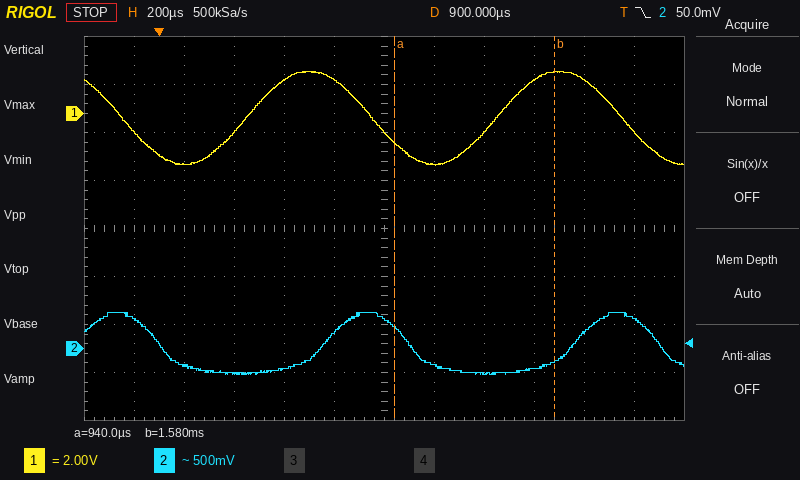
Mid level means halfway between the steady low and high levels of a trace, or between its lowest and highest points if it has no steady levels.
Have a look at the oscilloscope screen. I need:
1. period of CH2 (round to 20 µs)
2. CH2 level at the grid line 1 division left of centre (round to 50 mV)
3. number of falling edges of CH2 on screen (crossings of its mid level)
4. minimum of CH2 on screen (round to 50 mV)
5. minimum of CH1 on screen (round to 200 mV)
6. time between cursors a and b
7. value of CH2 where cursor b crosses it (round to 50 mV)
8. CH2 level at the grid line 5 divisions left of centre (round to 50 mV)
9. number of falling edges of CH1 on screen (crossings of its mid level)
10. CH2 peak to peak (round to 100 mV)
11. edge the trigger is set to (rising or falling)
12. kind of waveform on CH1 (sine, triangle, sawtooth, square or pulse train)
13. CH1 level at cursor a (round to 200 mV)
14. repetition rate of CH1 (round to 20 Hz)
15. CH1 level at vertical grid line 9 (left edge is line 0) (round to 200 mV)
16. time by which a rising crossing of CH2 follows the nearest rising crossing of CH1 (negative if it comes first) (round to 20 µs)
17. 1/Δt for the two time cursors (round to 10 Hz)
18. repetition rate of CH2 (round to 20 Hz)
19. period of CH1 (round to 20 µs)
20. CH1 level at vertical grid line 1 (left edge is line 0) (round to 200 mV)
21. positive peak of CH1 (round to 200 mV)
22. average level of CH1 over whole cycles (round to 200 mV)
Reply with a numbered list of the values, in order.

1. 1.00 ms
2. 150 mV
3. 3
4. -250 mV
5. -2.2 V
6. 640 µs
7. -150 mV
8. 300 mV
9. 3
10. 600 mV
11. falling
12. sine
13. -1.2 V
14. 1.00 kHz
15. 1.4 V
16. +320 µs
17. 1.56 kHz
18. 1.00 kHz
19. 1.00 ms
20. -800 mV
21. 1.8 V
22. -200 mV
